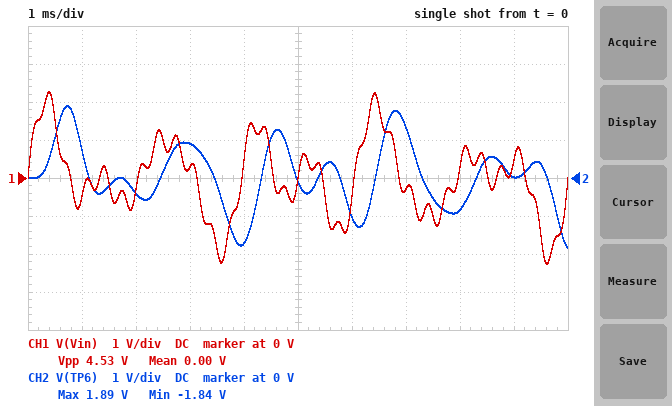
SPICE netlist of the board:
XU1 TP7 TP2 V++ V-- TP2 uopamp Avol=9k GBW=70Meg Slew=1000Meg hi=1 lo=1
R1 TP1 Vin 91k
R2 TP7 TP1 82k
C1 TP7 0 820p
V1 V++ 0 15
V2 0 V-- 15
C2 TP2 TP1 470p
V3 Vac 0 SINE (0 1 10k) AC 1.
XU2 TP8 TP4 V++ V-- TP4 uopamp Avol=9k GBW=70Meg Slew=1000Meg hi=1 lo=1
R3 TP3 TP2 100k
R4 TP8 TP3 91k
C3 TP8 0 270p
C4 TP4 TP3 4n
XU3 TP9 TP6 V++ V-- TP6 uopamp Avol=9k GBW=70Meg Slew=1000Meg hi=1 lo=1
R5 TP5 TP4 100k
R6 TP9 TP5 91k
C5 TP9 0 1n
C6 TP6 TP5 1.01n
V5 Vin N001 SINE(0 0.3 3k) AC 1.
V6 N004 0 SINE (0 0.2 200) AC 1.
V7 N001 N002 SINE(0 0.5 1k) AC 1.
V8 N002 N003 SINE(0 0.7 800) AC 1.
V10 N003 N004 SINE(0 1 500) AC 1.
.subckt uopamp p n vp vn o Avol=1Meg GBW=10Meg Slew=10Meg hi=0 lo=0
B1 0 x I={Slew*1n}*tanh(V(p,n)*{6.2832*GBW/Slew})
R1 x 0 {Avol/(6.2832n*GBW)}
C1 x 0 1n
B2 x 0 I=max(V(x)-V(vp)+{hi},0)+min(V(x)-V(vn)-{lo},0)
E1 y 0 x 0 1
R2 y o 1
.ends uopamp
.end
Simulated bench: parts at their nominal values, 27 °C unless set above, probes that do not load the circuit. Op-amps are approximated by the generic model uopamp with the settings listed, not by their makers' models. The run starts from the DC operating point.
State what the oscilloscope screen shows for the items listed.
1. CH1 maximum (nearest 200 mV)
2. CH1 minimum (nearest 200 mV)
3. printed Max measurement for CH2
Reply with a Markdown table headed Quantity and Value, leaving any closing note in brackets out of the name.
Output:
| Quantity | Value |
|---|---|
| CH1 maximum | 2.2 V |
| CH1 minimum | -2.2 V |
| printed Max measurement for CH2 | 1.89 V |
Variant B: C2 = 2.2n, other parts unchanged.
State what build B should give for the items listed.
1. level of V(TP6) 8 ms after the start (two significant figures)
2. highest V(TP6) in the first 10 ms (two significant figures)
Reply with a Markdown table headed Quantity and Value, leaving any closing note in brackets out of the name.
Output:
| Quantity | Value |
|---|---|
| level of V(TP6) 8 ms after the start | -920 mV |
| highest V(TP6) in the first 10 ms | 2.1 V |
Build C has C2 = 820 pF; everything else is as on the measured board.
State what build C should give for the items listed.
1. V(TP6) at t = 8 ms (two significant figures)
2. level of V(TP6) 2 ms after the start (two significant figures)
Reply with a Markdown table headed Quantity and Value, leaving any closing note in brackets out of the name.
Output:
| Quantity | Value |
|---|---|
| V(TP6) at t = 8 ms | -860 mV |
| level of V(TP6) 2 ms after the start | -400 mV |
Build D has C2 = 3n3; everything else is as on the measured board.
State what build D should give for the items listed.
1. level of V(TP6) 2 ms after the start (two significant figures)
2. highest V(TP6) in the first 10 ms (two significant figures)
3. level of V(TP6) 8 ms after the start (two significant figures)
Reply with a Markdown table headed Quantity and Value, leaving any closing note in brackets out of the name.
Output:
| Quantity | Value |
|---|---|
| level of V(TP6) 2 ms after the start | -170 mV |
| highest V(TP6) in the first 10 ms | 2.3 V |
| level of V(TP6) 8 ms after the start | -950 mV |
